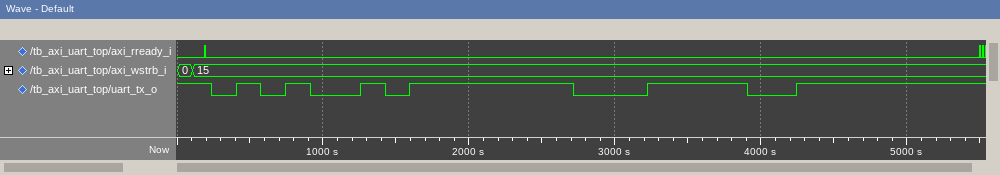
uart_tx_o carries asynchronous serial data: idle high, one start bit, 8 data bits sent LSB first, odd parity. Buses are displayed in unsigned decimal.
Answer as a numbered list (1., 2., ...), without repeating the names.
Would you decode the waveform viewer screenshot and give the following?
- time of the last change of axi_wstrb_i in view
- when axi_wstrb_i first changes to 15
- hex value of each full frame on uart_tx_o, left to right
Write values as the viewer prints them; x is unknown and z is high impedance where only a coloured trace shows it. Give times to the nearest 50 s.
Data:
1. 100 s
2. 100 s
3. A5, 3C
